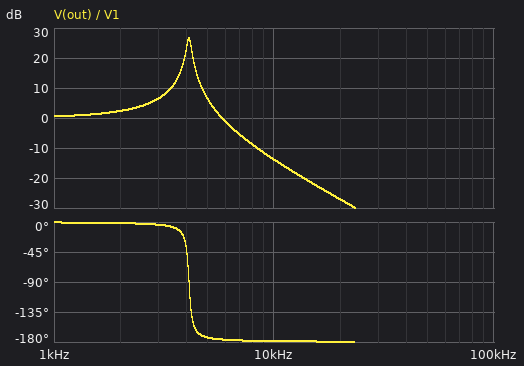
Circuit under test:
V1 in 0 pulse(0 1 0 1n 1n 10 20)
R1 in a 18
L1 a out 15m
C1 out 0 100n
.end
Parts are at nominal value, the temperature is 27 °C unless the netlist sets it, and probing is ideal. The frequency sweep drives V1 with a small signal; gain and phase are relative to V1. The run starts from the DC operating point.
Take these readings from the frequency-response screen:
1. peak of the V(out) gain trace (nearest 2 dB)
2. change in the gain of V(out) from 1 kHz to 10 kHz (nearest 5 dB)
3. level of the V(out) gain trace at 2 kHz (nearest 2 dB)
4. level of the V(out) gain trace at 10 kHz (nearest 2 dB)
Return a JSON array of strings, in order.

["26 dB", "-15 dB", "2 dB", "-14 dB"]
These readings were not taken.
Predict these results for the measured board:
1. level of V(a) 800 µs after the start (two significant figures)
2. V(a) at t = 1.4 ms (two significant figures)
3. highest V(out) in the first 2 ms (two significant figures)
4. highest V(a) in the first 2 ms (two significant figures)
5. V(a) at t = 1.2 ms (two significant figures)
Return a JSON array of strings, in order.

["970 mV", "1.0 V", "1.9 V", "1.0 V", "1.0 V"]
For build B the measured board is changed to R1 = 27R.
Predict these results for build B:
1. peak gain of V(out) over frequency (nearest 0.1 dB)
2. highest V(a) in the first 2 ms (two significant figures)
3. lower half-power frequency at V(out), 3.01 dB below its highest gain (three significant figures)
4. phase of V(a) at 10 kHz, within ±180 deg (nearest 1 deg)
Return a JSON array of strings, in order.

["23.1 dB", "1.1 V", "3.96 kHz", "2 deg"]
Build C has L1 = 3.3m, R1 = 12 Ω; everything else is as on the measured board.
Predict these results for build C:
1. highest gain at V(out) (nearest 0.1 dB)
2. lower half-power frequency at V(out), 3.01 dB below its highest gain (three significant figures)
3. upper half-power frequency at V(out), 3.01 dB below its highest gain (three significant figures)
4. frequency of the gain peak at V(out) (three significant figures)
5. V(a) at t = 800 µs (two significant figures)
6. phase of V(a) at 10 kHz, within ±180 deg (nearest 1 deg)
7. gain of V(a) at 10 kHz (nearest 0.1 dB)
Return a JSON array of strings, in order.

["23.6 dB", "8.46 kHz", "9.04 kHz", "8.75 kHz", "1.0 V", "14 deg", "-0.3 dB"]
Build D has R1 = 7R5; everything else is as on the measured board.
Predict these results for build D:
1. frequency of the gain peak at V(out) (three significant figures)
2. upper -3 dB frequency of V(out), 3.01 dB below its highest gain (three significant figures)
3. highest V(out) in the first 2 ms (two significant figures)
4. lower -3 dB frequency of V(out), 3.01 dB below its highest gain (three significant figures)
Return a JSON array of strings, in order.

["4.11 kHz", "4.15 kHz", "2.0 V", "4.07 kHz"]
